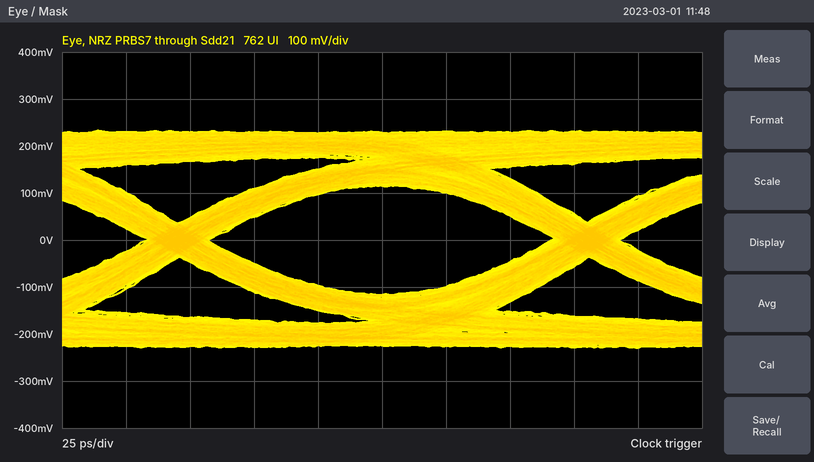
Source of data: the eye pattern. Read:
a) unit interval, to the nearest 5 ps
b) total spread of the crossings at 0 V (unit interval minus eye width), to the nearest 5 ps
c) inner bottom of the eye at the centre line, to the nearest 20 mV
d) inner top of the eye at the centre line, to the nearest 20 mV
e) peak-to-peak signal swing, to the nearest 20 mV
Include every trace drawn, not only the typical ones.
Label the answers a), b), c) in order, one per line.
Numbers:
a) 160 ps
b) 25 ps
c) -120 mV
d) 120 mV
e) 460 mV
